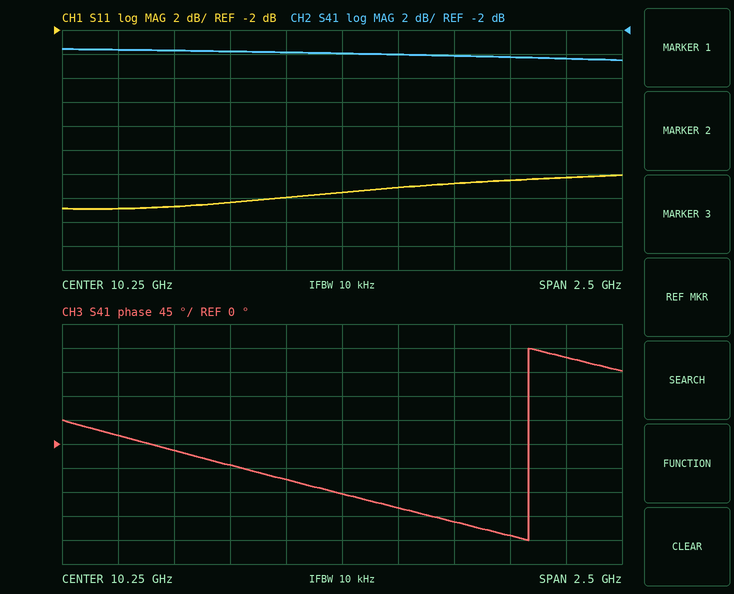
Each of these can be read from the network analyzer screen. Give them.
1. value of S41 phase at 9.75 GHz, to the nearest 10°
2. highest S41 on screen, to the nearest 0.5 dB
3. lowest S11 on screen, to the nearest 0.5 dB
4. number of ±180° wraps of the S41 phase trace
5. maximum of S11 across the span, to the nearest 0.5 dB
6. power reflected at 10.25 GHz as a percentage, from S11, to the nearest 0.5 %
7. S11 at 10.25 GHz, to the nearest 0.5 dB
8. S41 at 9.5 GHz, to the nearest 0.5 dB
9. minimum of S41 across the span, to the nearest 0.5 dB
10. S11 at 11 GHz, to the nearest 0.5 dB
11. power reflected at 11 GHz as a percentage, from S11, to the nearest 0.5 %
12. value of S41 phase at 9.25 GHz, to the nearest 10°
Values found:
-40°
-3.5 dB
-17.0 dB
1
-14.0 dB
3.0 %
-15.5 dB
-3.5 dB
-4.5 dB
-14.5 dB
3.5 %
20°
